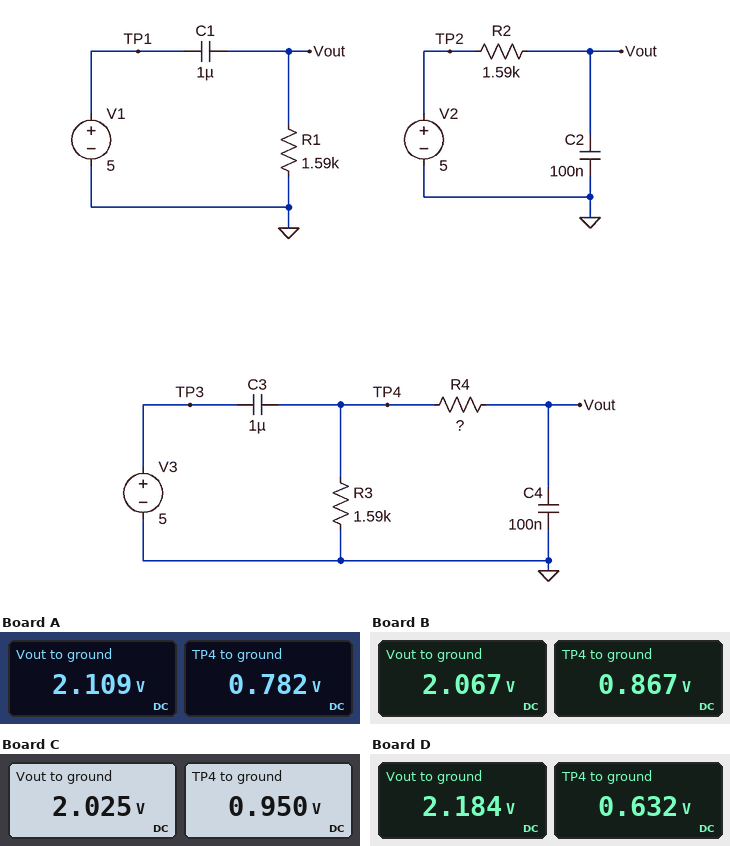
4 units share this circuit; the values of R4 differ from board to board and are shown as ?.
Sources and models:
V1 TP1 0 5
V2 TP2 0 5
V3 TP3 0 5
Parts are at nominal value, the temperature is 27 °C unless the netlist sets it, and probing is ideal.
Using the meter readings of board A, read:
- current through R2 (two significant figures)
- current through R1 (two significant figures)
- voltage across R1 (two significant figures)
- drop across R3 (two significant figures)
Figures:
1.8 mA
1.3 mA
2.1 V
780 mV
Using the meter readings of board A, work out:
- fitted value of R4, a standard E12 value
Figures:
2.7 kΩ
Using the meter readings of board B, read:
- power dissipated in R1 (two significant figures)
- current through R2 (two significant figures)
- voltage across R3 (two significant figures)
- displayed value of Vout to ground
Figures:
2.7 mW
1.8 mA
870 mV
2.067 V
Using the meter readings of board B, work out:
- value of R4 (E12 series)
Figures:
2.2 kΩ
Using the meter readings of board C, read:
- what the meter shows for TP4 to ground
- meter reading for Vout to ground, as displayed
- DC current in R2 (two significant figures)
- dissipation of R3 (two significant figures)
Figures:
0.950 V
2.025 V
1.9 mA
570 µW
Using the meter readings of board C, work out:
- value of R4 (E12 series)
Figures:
1.8 kΩ
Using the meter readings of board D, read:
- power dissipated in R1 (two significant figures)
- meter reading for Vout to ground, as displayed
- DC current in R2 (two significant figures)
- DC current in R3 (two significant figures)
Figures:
3.0 mW
2.184 V
1.8 mA
400 µA
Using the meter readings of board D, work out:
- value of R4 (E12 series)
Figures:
3.9 kΩ
